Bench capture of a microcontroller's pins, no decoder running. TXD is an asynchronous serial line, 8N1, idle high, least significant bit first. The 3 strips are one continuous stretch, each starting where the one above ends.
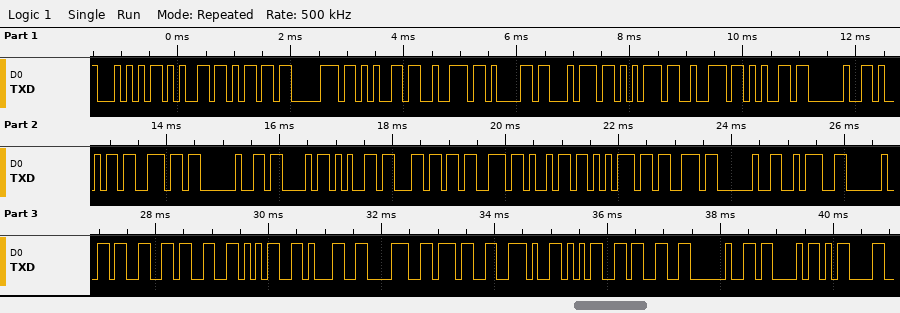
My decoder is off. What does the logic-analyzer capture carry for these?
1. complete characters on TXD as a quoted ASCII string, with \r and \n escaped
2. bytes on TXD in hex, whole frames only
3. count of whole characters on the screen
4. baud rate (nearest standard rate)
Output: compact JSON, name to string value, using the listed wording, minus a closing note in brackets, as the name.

{"complete characters on TXD as a quoted ASCII string, with \\r and \\n escaped": "\"Temperature in Celsius : 335187.53 C\\r\"", "bytes on TXD in hex, whole frames only": "0x54 0x65 0x6D 0x70 0x65 0x72 0x61 0x74 0x75 0x72 0x65 0x20 0x69 0x6E 0x20 0x43 0x65 0x6C 0x73 0x69 0x75 0x73 0x20 0x3A 0x20 0x33 0x33 0x35 0x31 0x38 0x37 0x2E 0x35 0x33 0x20 0x43 0x0D", "count of whole characters on the screen": "37", "baud rate": "9600 baud"}
